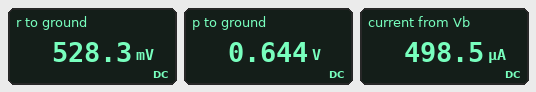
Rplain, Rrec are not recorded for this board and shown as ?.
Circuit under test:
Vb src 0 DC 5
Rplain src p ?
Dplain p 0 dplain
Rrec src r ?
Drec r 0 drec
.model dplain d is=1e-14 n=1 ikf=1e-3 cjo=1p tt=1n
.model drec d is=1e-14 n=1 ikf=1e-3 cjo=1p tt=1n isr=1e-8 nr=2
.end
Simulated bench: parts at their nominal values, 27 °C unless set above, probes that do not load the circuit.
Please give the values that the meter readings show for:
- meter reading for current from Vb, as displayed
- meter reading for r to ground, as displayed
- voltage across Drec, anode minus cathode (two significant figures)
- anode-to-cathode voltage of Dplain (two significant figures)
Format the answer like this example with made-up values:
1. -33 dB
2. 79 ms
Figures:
1. 498.5 µA
2. 528.3 mV
3. 530 mV
4. 640 mV
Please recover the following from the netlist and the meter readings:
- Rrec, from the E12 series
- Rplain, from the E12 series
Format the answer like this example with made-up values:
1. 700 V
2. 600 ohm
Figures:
1. 33 kΩ
2. 12 kΩ
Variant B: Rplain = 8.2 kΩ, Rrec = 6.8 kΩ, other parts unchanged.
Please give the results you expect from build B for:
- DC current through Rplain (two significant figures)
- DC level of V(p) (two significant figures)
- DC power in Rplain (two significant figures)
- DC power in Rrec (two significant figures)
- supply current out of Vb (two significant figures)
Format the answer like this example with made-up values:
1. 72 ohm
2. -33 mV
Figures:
1. 530 µA
2. 660 mV
3. 2.3 mW
4. 2.8 mW
5. 1.2 mA
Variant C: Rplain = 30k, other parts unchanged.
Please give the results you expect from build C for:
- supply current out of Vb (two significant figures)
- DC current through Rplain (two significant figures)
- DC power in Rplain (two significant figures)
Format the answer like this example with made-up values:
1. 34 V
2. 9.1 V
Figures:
1. 280 µA
2. 150 µA
3. 640 µW
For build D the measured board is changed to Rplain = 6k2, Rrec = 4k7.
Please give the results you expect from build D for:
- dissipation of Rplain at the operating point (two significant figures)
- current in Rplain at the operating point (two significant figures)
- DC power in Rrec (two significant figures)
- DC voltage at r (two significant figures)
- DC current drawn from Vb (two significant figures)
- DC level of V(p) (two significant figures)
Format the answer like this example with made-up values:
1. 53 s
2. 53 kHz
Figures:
1. 3.0 mW
2. 700 µA
3. 4.0 mW
4. 650 mV
5. 1.6 mA
6. 670 mV
